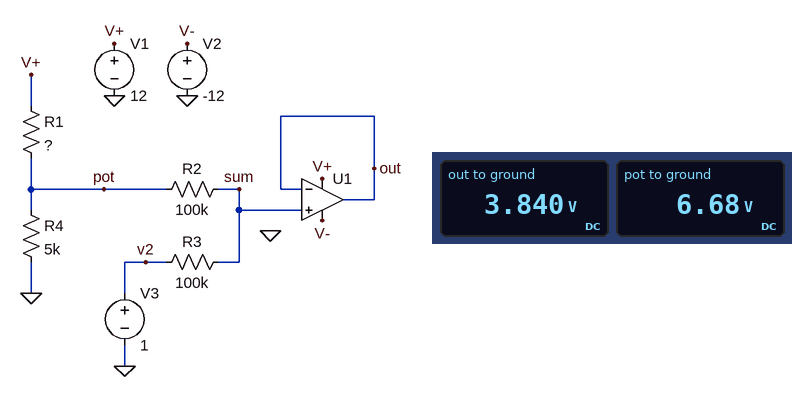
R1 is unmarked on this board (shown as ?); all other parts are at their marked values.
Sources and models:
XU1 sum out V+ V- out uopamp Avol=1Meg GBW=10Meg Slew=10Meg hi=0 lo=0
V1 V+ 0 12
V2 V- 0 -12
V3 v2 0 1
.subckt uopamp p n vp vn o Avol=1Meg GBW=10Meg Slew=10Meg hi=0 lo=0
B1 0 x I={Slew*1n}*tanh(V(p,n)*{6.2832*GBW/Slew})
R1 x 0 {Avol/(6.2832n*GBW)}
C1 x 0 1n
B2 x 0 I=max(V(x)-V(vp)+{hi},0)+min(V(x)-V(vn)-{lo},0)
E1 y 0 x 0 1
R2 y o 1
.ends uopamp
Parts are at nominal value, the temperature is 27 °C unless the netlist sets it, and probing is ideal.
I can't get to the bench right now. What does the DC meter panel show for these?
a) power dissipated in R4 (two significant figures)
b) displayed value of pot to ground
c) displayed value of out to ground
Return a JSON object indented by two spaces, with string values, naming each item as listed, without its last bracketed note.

{
  "power dissipated in R4": "8.9 mW",
  "displayed value of pot to ground": "6.68 V",
  "displayed value of out to ground": "3.840 V"
}
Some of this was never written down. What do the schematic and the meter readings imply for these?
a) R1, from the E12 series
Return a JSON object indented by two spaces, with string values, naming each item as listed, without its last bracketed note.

{
  "R1, from the E12 series": "3.9 kΩ"
}
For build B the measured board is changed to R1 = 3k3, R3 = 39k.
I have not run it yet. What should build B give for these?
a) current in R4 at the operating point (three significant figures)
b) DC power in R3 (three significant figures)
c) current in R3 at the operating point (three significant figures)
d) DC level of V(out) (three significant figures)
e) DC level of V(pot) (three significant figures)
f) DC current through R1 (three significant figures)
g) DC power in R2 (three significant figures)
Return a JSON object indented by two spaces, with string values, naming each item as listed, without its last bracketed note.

{
  "current in R4 at the operating point": "1.43 mA",
  "DC power in R3": "76.1 µW",
  "current in R3 at the operating point": "44.2 µA",
  "DC level of V(out)": "2.72 V",
  "DC level of V(pot)": "7.14 V",
  "DC current through R1": "1.47 mA",
  "DC power in R2": "195 µW"
}
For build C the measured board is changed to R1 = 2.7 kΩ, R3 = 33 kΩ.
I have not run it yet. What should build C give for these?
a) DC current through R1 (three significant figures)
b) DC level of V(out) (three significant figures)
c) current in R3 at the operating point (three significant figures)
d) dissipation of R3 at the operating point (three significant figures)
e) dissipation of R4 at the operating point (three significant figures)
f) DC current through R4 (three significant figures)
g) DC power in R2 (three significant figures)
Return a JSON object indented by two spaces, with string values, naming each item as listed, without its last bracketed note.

{
  "DC current through R1": "1.59 mA",
  "DC level of V(out)": "2.66 V",
  "current in R3 at the operating point": "50.4 µA",
  "dissipation of R3 at the operating point": "83.8 µW",
  "dissipation of R4 at the operating point": "11.9 mW",
  "DC current through R4": "1.54 mA",
  "DC power in R2": "254 µW"
}
